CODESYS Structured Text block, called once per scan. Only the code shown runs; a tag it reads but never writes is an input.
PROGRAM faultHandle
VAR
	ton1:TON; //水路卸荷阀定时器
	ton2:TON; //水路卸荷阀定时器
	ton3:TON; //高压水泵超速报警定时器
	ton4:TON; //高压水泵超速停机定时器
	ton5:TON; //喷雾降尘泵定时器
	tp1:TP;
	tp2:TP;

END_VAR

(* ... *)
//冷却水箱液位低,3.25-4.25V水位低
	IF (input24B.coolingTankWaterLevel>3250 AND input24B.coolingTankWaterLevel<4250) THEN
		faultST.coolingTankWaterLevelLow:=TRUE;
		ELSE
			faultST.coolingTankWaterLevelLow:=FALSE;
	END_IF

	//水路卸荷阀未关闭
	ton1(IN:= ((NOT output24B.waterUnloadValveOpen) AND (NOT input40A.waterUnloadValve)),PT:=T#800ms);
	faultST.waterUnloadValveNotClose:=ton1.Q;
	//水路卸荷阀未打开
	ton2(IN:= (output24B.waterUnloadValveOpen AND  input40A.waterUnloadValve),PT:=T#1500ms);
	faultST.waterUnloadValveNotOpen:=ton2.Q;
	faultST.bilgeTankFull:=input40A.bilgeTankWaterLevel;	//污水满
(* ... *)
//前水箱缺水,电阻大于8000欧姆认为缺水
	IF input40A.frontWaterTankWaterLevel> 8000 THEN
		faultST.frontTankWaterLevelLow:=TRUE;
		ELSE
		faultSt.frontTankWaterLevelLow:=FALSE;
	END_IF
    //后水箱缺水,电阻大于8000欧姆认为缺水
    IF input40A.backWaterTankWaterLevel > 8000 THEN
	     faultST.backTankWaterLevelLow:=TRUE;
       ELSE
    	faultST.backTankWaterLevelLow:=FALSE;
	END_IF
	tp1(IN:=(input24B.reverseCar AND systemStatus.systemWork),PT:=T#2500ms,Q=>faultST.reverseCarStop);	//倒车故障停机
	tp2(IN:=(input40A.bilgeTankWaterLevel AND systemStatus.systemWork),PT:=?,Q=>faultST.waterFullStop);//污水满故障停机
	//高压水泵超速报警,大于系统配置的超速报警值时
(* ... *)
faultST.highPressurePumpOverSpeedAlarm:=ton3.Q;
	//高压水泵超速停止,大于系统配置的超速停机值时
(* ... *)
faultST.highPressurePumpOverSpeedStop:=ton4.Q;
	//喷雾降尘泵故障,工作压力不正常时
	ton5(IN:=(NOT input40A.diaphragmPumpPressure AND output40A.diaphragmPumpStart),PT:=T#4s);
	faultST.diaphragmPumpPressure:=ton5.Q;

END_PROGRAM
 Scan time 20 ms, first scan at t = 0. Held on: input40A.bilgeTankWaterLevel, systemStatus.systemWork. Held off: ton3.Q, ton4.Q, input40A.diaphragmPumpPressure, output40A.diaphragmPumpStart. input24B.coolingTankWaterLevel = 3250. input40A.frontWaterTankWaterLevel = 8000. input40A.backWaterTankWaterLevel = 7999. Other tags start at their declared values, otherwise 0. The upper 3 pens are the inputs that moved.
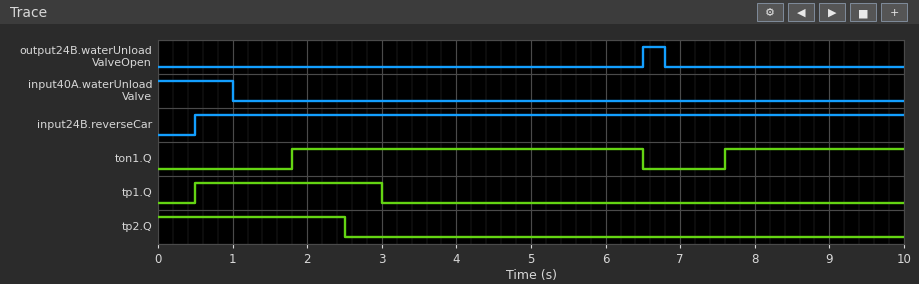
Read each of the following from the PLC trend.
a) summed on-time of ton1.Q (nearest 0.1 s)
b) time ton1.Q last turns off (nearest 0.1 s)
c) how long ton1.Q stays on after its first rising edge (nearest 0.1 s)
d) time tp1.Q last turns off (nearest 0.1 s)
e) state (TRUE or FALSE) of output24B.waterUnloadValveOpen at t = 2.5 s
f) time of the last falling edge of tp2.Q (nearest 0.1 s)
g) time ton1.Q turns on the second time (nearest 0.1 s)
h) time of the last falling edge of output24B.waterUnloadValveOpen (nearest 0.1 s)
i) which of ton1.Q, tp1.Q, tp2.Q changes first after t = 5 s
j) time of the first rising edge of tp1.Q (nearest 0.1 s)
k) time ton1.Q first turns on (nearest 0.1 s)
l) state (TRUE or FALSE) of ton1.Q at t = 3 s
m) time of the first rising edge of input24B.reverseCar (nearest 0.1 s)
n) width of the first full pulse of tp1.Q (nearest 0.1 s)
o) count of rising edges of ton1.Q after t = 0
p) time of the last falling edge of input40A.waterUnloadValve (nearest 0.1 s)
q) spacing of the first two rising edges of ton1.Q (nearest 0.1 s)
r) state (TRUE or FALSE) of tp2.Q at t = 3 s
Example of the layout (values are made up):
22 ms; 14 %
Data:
7.1 s; 6.5 s; 4.7 s; 3.0 s; FALSE; 2.5 s; 7.6 s; 6.8 s; ton1.Q; 0.5 s; 1.8 s; TRUE; 0.5 s; 2.5 s; 2; 1.0 s; 5.8 s; FALSE
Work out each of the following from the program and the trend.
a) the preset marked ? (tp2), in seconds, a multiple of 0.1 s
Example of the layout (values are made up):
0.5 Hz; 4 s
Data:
2.5 s
